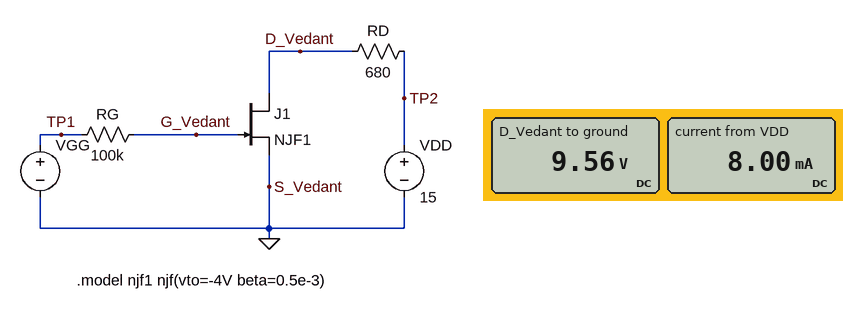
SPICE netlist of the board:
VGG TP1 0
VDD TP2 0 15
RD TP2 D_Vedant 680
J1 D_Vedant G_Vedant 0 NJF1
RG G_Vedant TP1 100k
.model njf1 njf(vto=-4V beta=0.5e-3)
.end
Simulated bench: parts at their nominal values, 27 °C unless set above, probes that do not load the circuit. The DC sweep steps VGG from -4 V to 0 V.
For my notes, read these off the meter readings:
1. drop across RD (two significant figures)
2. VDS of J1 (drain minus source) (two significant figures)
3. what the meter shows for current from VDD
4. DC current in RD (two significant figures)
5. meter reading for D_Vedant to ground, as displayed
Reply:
5.4 V
9.6 V
8.00 mA
8.0 mA
9.56 V
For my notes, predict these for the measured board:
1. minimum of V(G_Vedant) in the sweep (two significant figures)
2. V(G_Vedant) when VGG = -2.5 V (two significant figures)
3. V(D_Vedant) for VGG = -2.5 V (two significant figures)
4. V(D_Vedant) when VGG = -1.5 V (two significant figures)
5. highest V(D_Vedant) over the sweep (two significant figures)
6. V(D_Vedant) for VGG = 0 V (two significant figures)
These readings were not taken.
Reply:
-4.0 V
-2.5 V
14 V
13 V
15 V
9.6 V
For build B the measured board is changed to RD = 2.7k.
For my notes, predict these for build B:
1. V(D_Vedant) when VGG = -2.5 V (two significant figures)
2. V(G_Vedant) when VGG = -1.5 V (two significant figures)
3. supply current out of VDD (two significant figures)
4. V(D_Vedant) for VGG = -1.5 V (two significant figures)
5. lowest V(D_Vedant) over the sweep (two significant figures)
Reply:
12 V
-1.5 V
5.0 mA
6.6 V
1.5 V
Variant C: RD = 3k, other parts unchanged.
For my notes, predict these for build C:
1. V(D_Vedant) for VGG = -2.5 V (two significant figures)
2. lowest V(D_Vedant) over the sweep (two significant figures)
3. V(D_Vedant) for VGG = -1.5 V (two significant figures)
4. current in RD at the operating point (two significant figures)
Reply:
12 V
1.4 V
5.6 V
4.5 mA
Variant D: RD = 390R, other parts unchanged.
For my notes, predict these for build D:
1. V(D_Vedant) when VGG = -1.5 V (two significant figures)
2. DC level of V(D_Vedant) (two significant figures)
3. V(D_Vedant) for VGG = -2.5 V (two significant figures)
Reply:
14 V
12 V
15 V
